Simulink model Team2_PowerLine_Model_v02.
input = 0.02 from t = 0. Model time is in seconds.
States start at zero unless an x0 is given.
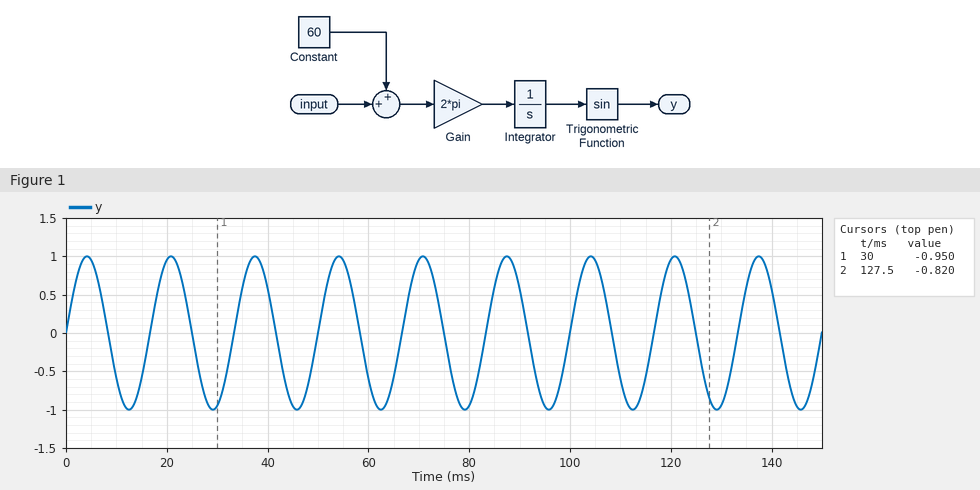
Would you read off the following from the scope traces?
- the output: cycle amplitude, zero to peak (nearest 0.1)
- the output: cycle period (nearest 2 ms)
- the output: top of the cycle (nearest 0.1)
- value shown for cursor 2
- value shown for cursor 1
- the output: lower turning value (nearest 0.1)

1.0
16 ms
1.0
-0.820
-0.950
-1.0
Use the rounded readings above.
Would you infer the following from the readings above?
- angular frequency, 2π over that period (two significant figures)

0.39 rad/ms
